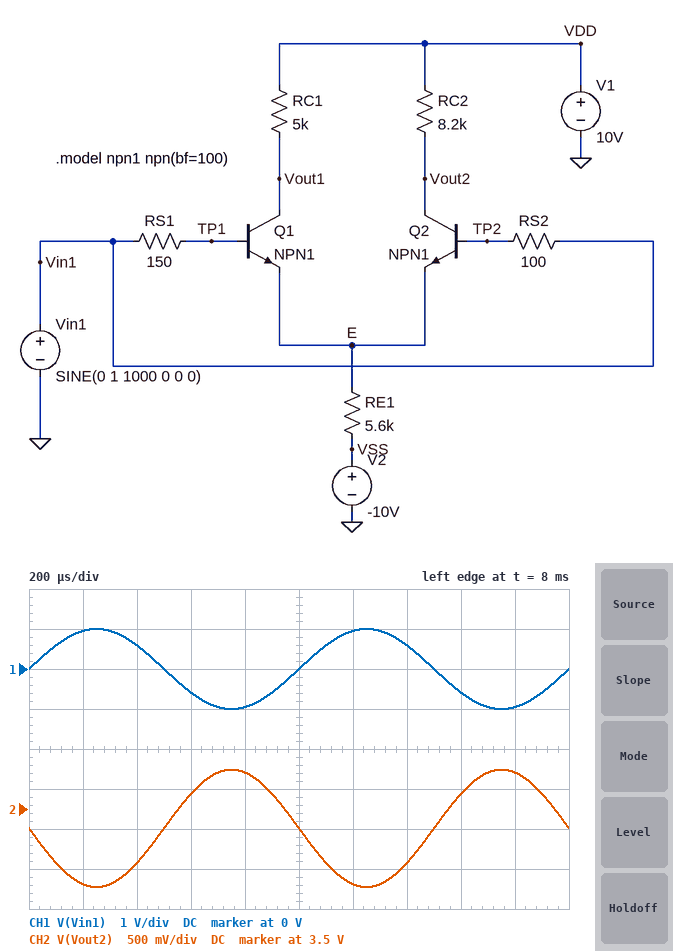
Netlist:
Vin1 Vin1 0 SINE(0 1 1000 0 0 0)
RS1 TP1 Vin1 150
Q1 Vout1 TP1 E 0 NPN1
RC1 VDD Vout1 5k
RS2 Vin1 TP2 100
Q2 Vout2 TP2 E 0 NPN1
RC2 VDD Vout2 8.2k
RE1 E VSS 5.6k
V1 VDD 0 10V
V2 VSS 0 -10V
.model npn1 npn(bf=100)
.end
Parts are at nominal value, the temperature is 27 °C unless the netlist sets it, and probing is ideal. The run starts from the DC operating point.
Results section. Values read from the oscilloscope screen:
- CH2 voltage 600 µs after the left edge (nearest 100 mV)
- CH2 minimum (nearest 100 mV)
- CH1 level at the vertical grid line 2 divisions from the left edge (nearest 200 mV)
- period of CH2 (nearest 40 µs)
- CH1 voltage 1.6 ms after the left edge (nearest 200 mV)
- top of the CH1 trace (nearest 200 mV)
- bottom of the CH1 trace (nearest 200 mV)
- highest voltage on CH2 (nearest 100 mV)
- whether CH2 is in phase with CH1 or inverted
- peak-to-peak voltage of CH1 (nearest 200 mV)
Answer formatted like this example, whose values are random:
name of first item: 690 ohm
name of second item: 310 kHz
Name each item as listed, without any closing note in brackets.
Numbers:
CH2 voltage 600 µs after the left edge: 3.7 V
CH2 minimum: 2.5 V
CH1 level at the vertical grid line 2 divisions from the left edge: 600 mV
period of CH2: 1.00 ms
CH1 voltage 1.6 ms after the left edge: -600 mV
top of the CH1 trace: 1.0 V
bottom of the CH1 trace: -1.0 V
highest voltage on CH2: 4.0 V
whether CH2 is in phase with CH1 or inverted: inverted
peak-to-peak voltage of CH1: 2.0 V
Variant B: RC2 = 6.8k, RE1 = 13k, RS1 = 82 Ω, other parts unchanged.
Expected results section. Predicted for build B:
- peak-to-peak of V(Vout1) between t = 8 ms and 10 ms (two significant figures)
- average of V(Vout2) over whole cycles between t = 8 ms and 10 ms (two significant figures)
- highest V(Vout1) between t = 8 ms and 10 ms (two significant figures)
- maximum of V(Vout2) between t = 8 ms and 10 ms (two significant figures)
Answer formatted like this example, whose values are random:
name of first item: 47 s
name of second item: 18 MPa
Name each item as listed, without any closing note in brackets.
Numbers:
peak-to-peak of V(Vout1) between t = 8 ms and 10 ms: 380 mV
average of V(Vout2) over whole cycles between t = 8 ms and 10 ms: 7.6 V
highest V(Vout1) between t = 8 ms and 10 ms: 8.4 V
maximum of V(Vout2) between t = 8 ms and 10 ms: 7.9 V
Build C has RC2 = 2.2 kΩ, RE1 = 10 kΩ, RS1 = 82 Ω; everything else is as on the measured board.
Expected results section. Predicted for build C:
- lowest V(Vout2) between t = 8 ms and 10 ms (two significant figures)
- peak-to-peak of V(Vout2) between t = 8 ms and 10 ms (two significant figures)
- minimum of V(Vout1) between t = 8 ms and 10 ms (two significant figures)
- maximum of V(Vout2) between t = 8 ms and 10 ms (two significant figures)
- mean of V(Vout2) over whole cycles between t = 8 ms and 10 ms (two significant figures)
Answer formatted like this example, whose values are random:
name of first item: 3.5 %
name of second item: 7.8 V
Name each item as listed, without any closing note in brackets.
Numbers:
lowest V(Vout2) between t = 8 ms and 10 ms: 8.9 V
peak-to-peak of V(Vout2) between t = 8 ms and 10 ms: 220 mV
minimum of V(Vout1) between t = 8 ms and 10 ms: 7.5 V
maximum of V(Vout2) between t = 8 ms and 10 ms: 9.1 V
mean of V(Vout2) over whole cycles between t = 8 ms and 10 ms: 9.0 V
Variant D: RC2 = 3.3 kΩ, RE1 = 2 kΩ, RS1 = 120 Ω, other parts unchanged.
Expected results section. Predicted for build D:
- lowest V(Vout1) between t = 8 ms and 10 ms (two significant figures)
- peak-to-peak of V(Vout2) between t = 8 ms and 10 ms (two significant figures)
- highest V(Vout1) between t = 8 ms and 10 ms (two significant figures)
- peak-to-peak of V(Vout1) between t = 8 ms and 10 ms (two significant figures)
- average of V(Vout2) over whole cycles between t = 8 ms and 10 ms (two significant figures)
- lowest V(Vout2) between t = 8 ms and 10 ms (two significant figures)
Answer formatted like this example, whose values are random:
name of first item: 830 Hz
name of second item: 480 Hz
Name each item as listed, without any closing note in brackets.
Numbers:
lowest V(Vout1) between t = 8 ms and 10 ms: -900 mV
peak-to-peak of V(Vout2) between t = 8 ms and 10 ms: 3.0 V
highest V(Vout1) between t = 8 ms and 10 ms: 270 mV
peak-to-peak of V(Vout1) between t = 8 ms and 10 ms: 1.2 V
average of V(Vout2) over whole cycles between t = 8 ms and 10 ms: 1.9 V
lowest V(Vout2) between t = 8 ms and 10 ms: 260 mV
